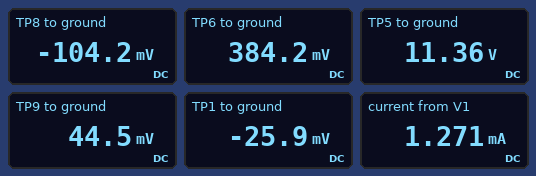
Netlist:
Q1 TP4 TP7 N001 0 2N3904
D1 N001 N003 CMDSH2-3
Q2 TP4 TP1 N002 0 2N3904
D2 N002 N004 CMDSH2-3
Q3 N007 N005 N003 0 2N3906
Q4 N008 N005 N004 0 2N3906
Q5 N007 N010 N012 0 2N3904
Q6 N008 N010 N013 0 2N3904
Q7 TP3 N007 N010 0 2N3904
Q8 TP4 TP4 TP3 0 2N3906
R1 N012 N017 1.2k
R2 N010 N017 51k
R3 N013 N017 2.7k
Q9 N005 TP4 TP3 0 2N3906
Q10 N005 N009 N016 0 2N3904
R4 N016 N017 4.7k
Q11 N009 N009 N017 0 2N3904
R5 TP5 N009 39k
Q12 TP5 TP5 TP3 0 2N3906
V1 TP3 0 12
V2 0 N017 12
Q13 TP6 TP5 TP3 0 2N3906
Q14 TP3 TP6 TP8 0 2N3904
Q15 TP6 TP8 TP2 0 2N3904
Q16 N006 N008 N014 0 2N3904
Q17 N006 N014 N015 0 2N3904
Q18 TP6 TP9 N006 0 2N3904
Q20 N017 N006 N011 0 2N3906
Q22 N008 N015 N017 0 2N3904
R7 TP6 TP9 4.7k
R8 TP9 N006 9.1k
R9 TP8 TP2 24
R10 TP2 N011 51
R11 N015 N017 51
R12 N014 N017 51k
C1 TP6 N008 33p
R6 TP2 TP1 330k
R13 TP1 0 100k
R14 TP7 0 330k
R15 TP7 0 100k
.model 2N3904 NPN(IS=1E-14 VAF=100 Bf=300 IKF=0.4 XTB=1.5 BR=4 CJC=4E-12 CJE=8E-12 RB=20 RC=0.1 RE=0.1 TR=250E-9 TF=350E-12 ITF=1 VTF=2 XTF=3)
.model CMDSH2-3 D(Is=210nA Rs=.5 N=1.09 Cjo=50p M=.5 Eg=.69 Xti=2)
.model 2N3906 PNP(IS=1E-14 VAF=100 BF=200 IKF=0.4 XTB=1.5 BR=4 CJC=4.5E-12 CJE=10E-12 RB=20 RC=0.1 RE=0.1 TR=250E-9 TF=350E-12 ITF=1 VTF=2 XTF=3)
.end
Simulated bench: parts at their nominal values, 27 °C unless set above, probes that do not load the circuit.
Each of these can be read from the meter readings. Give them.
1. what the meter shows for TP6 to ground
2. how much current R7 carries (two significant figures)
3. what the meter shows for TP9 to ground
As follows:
384.2 mV
72 µA
44.5 mV
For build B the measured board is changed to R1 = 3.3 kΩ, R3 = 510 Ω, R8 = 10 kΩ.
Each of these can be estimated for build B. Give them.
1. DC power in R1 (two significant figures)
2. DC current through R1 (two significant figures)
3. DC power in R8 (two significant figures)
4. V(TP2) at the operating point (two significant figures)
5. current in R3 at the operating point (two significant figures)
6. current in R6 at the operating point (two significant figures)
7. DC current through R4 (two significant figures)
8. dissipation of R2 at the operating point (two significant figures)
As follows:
130 nW
6.2 µA
41 µW
200 mV
11 µA
470 nA
19 µA
5.8 µW
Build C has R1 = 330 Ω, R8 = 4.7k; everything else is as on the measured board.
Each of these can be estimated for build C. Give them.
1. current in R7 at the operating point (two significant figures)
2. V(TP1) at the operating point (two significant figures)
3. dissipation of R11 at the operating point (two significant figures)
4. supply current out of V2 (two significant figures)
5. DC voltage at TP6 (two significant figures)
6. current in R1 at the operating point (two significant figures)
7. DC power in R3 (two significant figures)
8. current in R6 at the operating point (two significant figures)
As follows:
140 µA
-44 mV
20 µW
1.6 mA
450 mV
11 µA
110 nW
420 nA
